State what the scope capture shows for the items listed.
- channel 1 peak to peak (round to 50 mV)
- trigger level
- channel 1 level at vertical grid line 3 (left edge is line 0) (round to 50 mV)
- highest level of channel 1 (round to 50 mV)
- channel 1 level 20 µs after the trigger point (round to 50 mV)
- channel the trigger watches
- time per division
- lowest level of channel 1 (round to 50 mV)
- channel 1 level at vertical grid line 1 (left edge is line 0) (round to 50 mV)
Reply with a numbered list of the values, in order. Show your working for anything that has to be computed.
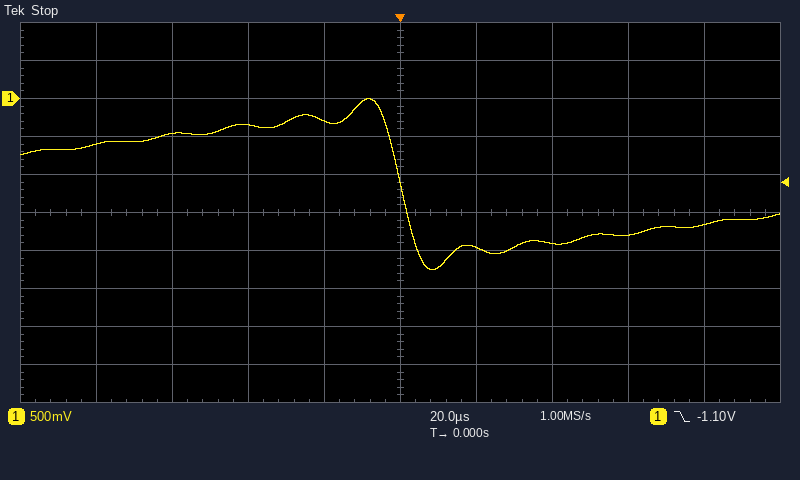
1. 0 mV − (-2.25 V) = 2.25 V
2. -1.10 V
3. -350 mV
4. 0 mV
5. -1.95 V
6. channel 1
7. 20 µs
8. -2.25 V
9. -600 mV
